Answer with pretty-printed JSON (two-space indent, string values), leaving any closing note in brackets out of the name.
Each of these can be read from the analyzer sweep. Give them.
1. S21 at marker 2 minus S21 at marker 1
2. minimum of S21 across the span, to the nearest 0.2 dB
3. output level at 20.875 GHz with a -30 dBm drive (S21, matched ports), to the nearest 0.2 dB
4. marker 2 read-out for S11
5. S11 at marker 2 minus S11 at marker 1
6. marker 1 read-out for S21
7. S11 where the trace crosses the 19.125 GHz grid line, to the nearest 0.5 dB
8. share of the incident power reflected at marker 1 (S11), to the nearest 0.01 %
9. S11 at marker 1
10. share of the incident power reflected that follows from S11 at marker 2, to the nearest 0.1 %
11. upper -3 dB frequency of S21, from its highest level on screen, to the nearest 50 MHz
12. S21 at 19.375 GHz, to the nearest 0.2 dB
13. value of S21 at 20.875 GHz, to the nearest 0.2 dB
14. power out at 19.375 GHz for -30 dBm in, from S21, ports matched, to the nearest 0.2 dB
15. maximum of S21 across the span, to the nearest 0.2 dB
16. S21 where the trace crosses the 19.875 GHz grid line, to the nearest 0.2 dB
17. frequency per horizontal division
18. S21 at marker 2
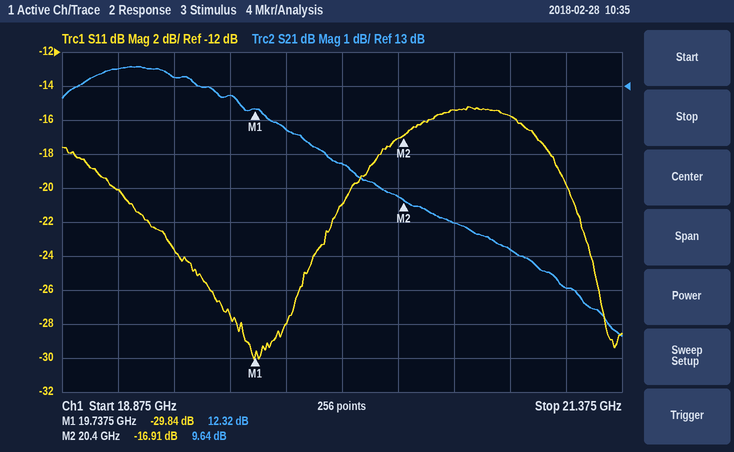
{
  "S21 at marker 2 minus S21 at marker 1": "-2.68 dB",
  "minimum of S21 across the span, to the nearest 0.2 dB": "5.6 dB",
  "output level at 20.875 GHz with a -30 dBm drive (S21, matched ports), to the nearest 0.2 dB": "-21.8 dBm",
  "marker 2 read-out for S11": "-16.91 dB",
  "S11 at marker 2 minus S11 at marker 1": "12.93 dB",
  "marker 1 read-out for S21": "12.32 dB",
  "S11 where the trace crosses the 19.125 GHz grid line, to the nearest 0.5 dB": "-20.0 dB",
  "share of the incident power reflected at marker 1 (S11), to the nearest 0.01 %": "0.10 %",
  "S11 at marker 1": "-29.84 dB",
  "share of the incident power reflected that follows from S11 at marker 2, to the nearest 0.1 %": "2.0 %",
  "upper -3 dB frequency of S21, from its highest level on screen, to the nearest 50 MHz": "20.15 GHz",
  "S21 at 19.375 GHz, to the nearest 0.2 dB": "13.2 dB",
  "value of S21 at 20.875 GHz, to the nearest 0.2 dB": "8.2 dB",
  "power out at 19.375 GHz for -30 dBm in, from S21, ports matched, to the nearest 0.2 dB": "-16.8 dBm",
  "maximum of S21 across the span, to the nearest 0.2 dB": "13.6 dB",
  "S21 where the trace crosses the 19.875 GHz grid line, to the nearest 0.2 dB": "11.8 dB",
  "frequency per horizontal division": "250 MHz",
  "S21 at marker 2": "9.64 dB"
}
